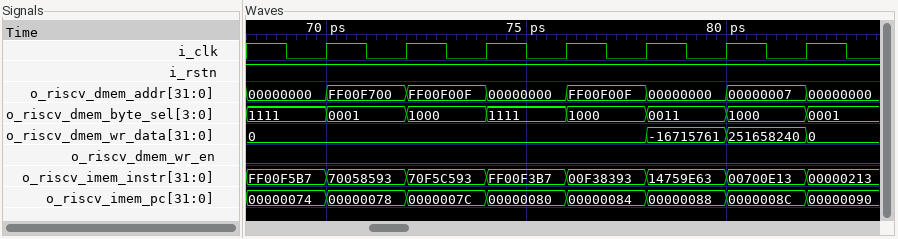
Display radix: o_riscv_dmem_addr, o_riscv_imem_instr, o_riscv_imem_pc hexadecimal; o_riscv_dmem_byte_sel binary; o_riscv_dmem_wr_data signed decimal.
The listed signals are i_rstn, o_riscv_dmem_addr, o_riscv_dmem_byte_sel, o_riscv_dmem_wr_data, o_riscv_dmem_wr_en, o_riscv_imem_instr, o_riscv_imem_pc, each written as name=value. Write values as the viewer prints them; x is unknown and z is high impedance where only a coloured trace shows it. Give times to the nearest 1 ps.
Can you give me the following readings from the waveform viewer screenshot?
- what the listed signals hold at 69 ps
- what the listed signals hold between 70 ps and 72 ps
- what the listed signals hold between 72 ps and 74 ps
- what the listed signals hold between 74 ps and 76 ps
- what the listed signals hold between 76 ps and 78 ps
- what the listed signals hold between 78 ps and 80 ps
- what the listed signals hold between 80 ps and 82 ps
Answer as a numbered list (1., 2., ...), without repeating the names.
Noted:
1. i_rstn=1, o_riscv_dmem_addr=00000000, o_riscv_dmem_byte_sel=1111, o_riscv_dmem_wr_data=0, o_riscv_dmem_wr_en=0, o_riscv_imem_instr=FF00F5B7, o_riscv_imem_pc=00000074
2. i_rstn=1, o_riscv_dmem_addr=FF00F700, o_riscv_dmem_byte_sel=0001, o_riscv_dmem_wr_data=0, o_riscv_dmem_wr_en=0, o_riscv_imem_instr=70058593, o_riscv_imem_pc=00000078
3. i_rstn=1, o_riscv_dmem_addr=FF00F00F, o_riscv_dmem_byte_sel=1000, o_riscv_dmem_wr_data=0, o_riscv_dmem_wr_en=0, o_riscv_imem_instr=70F5C593, o_riscv_imem_pc=0000007C
4. i_rstn=1, o_riscv_dmem_addr=00000000, o_riscv_dmem_byte_sel=1111, o_riscv_dmem_wr_data=0, o_riscv_dmem_wr_en=0, o_riscv_imem_instr=FF00F3B7, o_riscv_imem_pc=00000080
5. i_rstn=1, o_riscv_dmem_addr=FF00F00F, o_riscv_dmem_byte_sel=1000, o_riscv_dmem_wr_data=0, o_riscv_dmem_wr_en=0, o_riscv_imem_instr=00F38393, o_riscv_imem_pc=00000084
6. i_rstn=1, o_riscv_dmem_addr=00000000, o_riscv_dmem_byte_sel=0011, o_riscv_dmem_wr_data=-16715761, o_riscv_dmem_wr_en=0, o_riscv_imem_instr=14759E63, o_riscv_imem_pc=00000088
7. i_rstn=1, o_riscv_dmem_addr=00000007, o_riscv_dmem_byte_sel=1000, o_riscv_dmem_wr_data=251658240, o_riscv_dmem_wr_en=0, o_riscv_imem_instr=00700E13, o_riscv_imem_pc=0000008C
